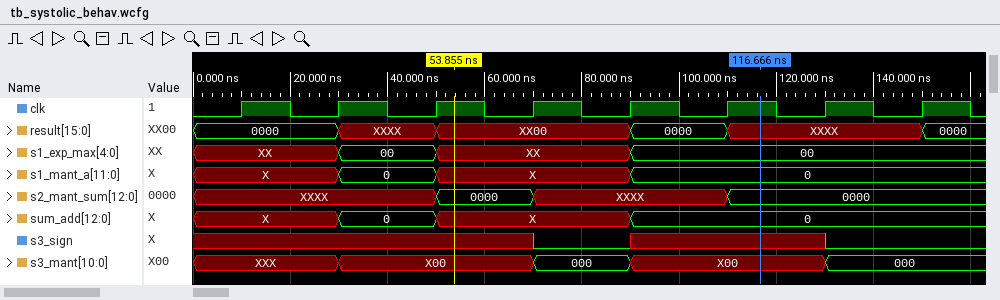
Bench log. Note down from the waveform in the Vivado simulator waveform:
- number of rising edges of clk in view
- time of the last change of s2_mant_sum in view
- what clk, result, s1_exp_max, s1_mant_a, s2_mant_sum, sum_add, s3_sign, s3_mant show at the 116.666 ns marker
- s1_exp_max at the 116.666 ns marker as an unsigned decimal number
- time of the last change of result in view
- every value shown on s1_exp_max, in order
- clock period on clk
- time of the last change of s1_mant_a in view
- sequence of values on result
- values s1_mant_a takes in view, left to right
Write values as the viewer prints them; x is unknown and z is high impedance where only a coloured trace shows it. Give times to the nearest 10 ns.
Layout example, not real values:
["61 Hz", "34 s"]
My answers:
["8", "110 ns", "clk=1, result=XXXX, s1_exp_max=00, s1_mant_a=0, s2_mant_sum=0000, sum_add=0, s3_sign=x, s3_mant=X00", "0", "150 ns", "XX, 00, XX, 00", "20 ns", "90 ns", "0000, XXXX, XX00, 0000, XXXX, 0000", "X, 0, X, 0"]
